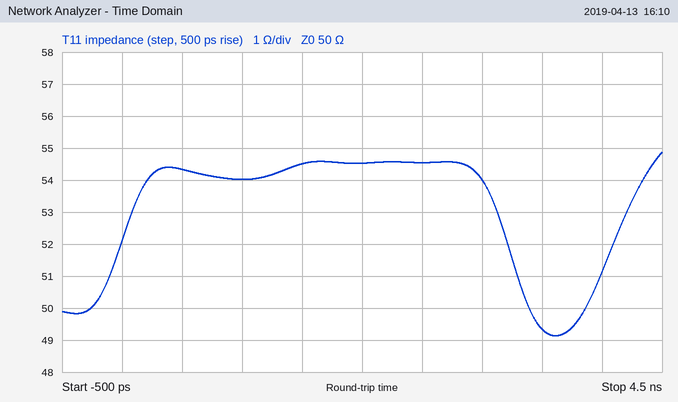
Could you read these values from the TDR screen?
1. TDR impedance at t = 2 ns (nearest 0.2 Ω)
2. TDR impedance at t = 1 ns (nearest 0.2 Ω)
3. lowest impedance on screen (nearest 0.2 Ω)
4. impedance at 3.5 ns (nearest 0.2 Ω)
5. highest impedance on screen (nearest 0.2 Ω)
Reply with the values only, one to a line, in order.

54.6 Ω
54.0 Ω
49.2 Ω
49.4 Ω
54.8 Ω
